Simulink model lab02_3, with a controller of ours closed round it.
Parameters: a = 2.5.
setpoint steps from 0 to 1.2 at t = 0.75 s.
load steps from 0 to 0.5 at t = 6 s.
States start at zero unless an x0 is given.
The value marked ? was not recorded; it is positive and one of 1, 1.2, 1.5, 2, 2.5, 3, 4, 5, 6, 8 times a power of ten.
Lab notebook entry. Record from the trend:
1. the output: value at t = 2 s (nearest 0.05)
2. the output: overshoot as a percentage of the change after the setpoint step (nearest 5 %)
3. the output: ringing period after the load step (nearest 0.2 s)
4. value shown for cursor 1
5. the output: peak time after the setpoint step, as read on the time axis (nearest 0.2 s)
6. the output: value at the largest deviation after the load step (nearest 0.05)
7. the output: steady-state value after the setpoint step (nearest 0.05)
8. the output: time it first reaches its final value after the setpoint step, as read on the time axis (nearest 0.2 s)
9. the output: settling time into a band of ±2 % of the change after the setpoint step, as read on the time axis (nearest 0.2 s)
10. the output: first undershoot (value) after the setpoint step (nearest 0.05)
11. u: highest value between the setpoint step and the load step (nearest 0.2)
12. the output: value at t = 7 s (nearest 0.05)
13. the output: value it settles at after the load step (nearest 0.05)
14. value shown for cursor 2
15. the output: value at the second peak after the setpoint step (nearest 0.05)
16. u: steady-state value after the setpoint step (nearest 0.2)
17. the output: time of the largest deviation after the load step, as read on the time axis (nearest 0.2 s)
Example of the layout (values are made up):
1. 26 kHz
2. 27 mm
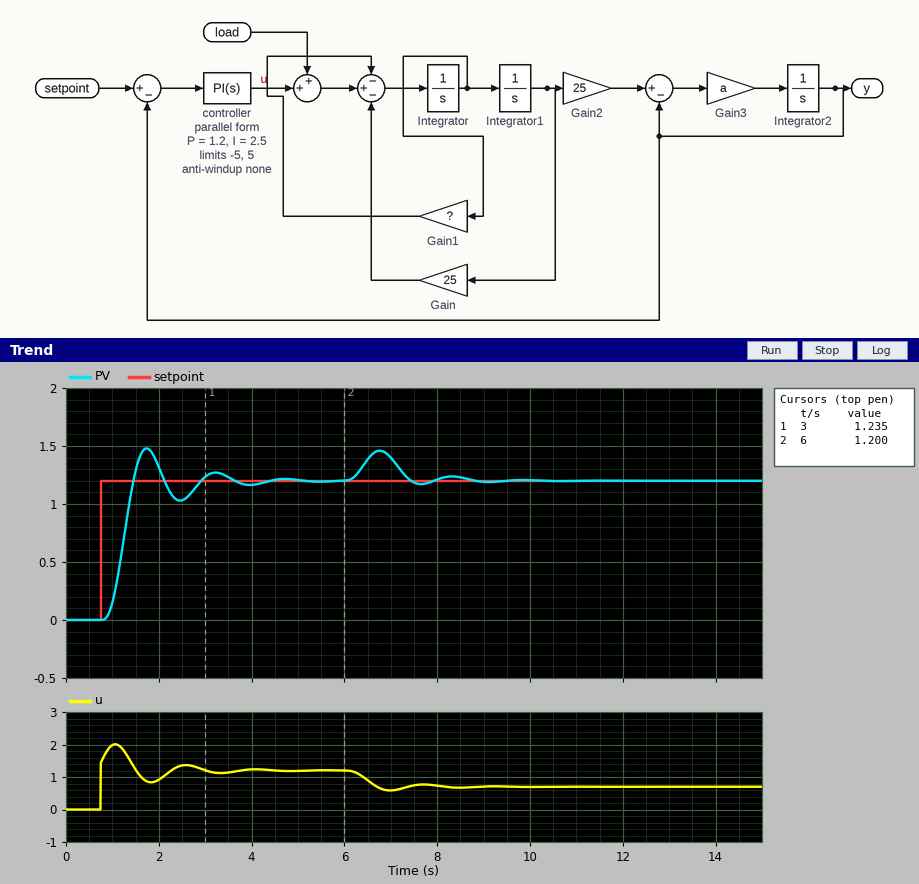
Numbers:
1. 1.30
2. 25 %
3. 1.6 s
4. 1.235
5. 1.8 s
6. 1.45
7. 1.20
8. 1.4 s
9. 4.2 s
10. 1.05
11. 2.0
12. 1.40
13. 1.20
14. 1.200
15. 1.25
16. 1.2
17. 6.8 s
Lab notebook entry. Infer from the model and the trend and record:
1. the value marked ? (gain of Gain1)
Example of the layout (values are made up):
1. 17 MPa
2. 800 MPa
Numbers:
1. 6
